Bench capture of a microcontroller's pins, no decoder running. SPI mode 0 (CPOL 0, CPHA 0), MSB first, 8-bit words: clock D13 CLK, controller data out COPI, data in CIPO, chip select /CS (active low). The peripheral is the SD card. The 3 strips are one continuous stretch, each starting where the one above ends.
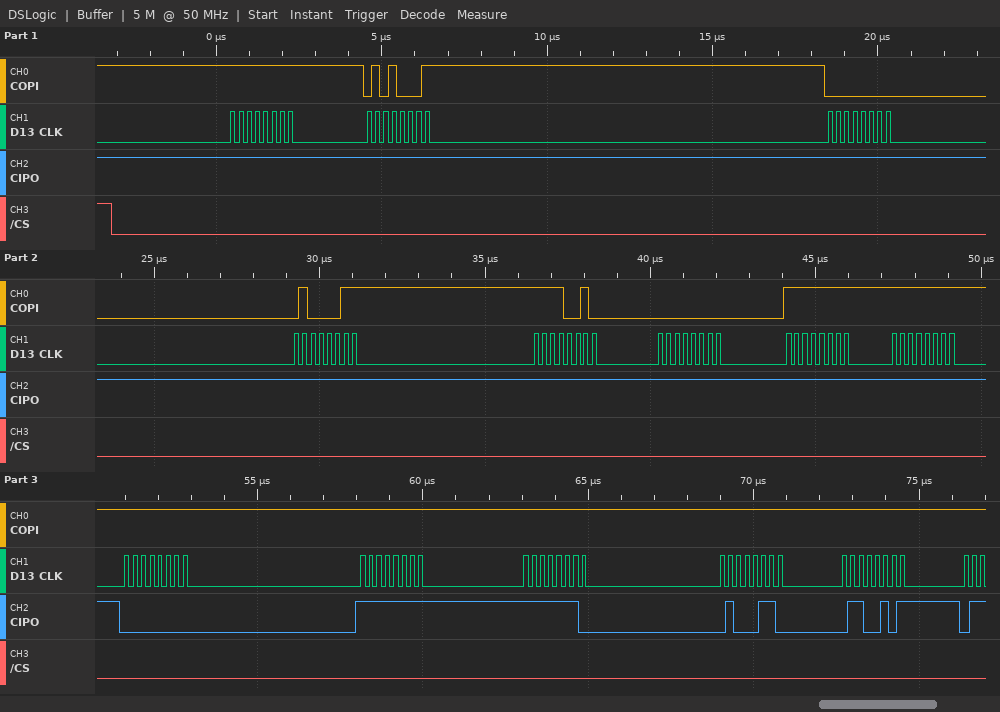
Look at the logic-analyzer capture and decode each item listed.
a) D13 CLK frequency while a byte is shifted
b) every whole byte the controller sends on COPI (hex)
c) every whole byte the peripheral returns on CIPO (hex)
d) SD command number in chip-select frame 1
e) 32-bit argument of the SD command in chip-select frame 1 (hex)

4 MHz
FF 51 00 43 F2 00 FF FF FF FF FF FF FF
FF FF FF FF FF FF FF FF 00 FF FE 46 65
CMD17
0x0043F200
